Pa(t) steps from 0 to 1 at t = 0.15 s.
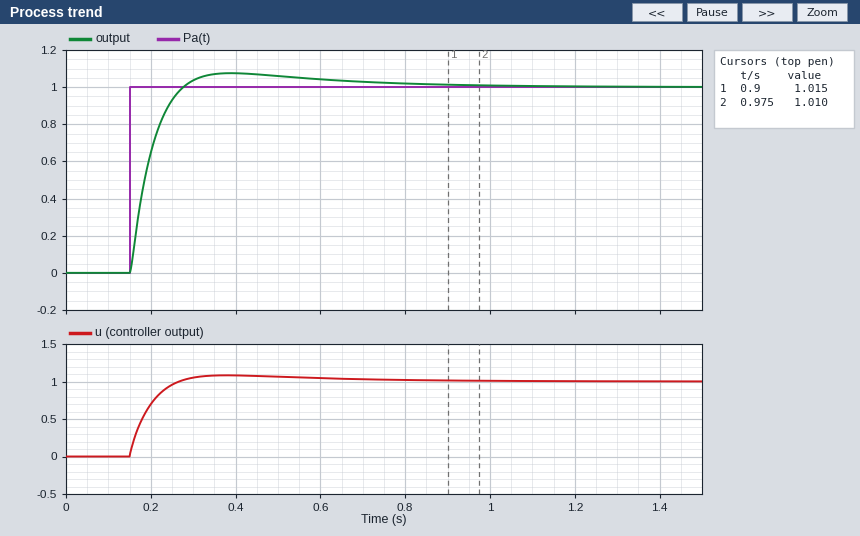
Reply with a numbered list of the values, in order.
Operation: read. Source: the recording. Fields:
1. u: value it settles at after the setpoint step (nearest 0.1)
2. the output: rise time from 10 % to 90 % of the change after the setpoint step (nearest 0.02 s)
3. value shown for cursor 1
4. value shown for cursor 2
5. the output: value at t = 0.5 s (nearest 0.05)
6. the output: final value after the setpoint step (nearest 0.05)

1. 1.0
2. 0.08 s
3. 1.015
4. 1.010
5. 1.05
6. 1.00
